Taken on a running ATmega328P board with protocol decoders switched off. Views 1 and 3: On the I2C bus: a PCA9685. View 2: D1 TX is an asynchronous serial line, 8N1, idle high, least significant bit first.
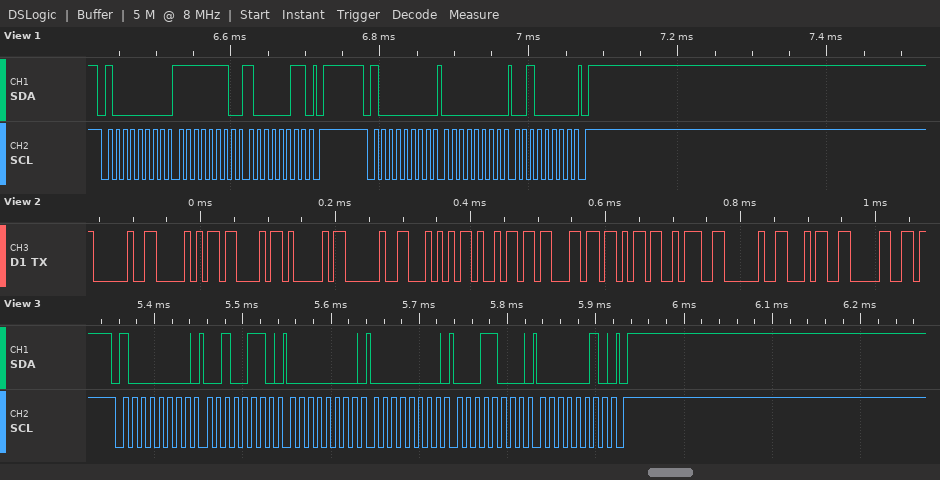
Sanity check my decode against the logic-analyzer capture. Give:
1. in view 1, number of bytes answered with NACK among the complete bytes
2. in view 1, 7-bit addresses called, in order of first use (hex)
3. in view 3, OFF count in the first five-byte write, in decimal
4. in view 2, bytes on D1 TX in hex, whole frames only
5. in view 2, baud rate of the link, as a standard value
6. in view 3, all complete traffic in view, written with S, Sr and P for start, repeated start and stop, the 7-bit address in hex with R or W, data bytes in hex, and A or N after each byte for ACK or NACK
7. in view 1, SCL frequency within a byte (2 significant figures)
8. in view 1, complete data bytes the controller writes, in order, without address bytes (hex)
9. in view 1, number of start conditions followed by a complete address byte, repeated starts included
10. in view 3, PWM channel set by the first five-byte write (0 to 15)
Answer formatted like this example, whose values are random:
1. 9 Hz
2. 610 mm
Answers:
1. 0
2. 0x40
3. 536
4. 0x20 0x50 0x43 0x41 0x20 0x54 0x69 0x63 0x6B 0x3A 0x20 0x34 0x30
5. 115200 baud
6. S 40W A 26 A 00 A 00 A 18 A 02 A P
7. 100 kHz
8. FE 83 00 20
9. 2
10. 8
